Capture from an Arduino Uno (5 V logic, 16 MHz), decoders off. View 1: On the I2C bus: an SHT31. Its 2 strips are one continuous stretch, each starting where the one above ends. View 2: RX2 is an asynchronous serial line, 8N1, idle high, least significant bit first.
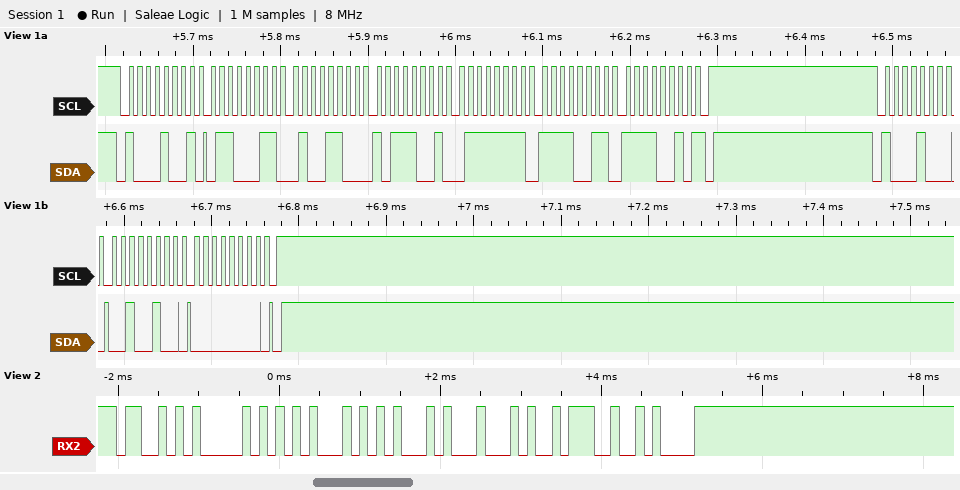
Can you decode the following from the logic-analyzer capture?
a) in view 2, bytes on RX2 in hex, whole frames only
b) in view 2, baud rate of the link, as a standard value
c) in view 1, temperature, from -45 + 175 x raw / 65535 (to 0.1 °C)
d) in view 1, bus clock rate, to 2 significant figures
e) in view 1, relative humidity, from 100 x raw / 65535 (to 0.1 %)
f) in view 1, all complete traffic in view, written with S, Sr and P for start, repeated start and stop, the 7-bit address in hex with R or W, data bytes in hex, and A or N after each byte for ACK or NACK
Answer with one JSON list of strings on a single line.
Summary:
["53 50 45 45 44 3A 0A", "9600 baud", "22.9 °C", "100 kHz", "50.0 %", "S 44R A 63 A 4C A B9 A 7F A F3 A F2 N P S 44W A 24 A 00 A P"]
